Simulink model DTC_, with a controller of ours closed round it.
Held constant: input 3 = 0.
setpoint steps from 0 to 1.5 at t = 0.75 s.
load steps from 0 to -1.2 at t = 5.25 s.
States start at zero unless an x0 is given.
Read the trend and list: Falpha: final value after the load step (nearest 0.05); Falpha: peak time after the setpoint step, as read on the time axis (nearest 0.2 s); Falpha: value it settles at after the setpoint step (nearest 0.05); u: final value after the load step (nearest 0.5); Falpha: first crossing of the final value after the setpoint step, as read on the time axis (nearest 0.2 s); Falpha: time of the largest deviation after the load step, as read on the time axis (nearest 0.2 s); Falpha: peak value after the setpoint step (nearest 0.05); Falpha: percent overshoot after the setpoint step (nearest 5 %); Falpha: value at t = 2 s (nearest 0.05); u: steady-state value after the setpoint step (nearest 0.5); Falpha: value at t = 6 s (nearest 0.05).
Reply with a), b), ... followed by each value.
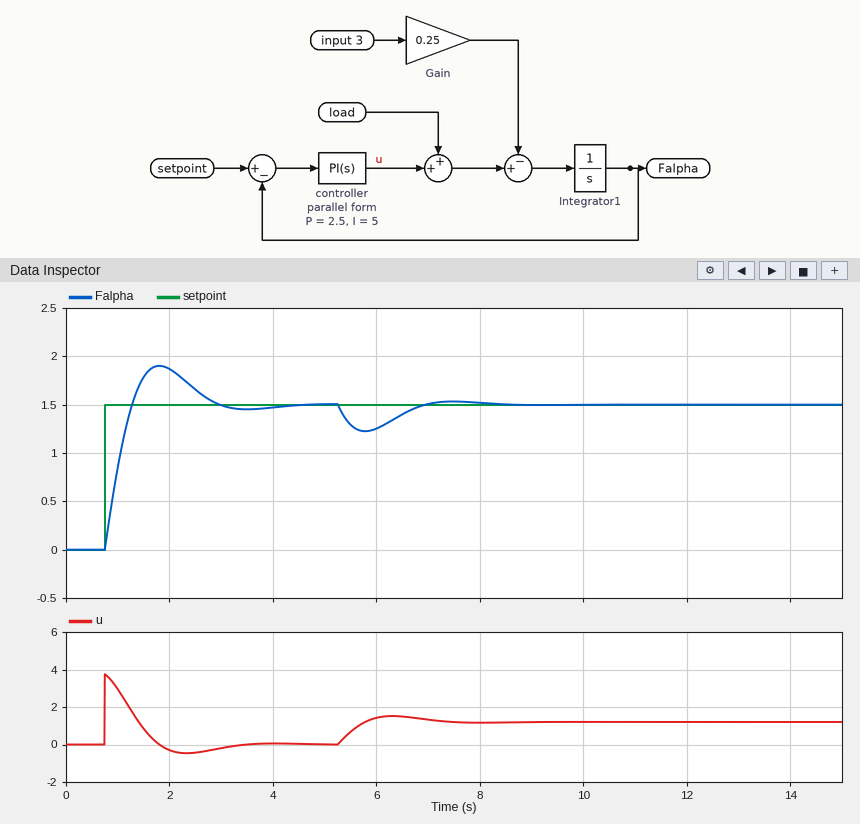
a) 1.50
b) 1.8 s
c) 1.50
d) 1.0
e) 1.2 s
f) 5.8 s
g) 1.90
h) 25 %
i) 1.85
j) 0.0
k) 1.25
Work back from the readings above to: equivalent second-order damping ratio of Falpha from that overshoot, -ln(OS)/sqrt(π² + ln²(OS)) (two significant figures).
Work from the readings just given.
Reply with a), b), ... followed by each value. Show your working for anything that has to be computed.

a) ln(0.25) = -1.386; 1.386 / sqrt(9.870 + 1.922) = 0.40
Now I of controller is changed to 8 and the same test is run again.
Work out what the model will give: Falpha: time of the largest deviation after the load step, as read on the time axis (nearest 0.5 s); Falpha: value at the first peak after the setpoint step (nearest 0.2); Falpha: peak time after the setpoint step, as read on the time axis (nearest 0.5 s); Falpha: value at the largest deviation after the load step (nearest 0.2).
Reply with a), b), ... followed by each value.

a) 5.5 s
b) 2.0
c) 1.5 s
d) 1.2
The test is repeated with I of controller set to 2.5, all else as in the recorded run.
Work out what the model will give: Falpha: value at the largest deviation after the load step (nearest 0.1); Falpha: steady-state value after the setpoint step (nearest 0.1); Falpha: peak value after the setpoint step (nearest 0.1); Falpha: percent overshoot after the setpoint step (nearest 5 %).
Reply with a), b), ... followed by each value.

a) 1.2
b) 1.5
c) 1.8
d) 20 %
